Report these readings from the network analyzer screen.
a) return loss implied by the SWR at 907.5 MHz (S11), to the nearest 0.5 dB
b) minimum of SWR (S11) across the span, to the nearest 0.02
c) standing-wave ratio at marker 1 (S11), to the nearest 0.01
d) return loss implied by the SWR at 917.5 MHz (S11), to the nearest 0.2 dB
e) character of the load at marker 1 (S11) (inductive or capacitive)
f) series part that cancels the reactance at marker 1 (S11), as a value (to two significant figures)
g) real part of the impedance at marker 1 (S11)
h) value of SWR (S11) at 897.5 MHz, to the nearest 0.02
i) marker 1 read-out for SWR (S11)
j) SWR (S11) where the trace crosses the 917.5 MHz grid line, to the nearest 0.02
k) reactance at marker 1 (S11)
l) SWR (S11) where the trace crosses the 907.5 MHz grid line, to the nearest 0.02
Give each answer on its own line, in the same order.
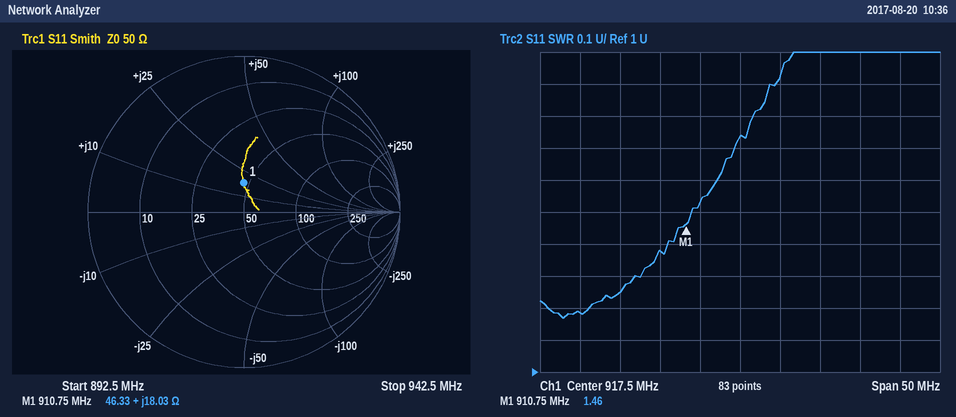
16.0 dB
1.16
1.46
11.4 dB
inductive
9.7 pF
46.33 Ω
1.18
1.46
1.74
+18.03 Ω
1.38
